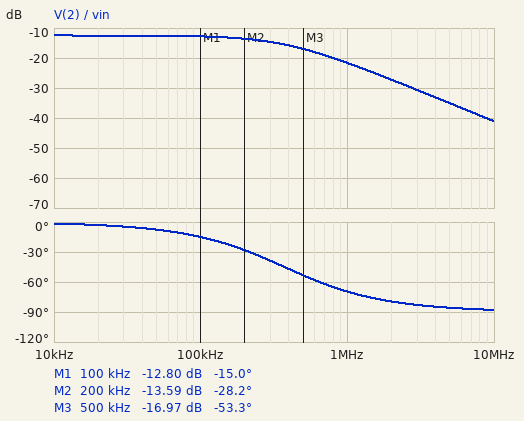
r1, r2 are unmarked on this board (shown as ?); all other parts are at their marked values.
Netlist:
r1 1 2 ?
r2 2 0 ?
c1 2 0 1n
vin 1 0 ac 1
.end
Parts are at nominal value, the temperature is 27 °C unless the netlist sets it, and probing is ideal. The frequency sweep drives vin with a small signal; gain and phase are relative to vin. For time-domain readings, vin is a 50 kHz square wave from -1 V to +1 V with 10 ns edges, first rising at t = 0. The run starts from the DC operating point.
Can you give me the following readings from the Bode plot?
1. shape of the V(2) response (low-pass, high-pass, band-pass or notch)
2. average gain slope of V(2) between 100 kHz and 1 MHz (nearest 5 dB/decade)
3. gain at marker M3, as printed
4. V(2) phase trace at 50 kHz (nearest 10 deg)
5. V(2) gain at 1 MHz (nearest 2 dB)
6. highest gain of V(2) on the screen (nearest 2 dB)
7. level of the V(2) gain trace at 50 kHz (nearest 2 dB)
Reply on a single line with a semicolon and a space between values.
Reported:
low-pass; -10 dB/decade; -16.97 dB; -10 deg; -22 dB; -12 dB; -12 dB
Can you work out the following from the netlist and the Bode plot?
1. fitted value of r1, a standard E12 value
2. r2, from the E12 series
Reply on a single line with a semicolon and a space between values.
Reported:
1.8 kΩ; 560 Ω
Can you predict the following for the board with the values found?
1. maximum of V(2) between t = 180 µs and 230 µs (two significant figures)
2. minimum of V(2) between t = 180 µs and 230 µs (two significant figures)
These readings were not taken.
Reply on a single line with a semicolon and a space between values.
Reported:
240 mV; -240 mV
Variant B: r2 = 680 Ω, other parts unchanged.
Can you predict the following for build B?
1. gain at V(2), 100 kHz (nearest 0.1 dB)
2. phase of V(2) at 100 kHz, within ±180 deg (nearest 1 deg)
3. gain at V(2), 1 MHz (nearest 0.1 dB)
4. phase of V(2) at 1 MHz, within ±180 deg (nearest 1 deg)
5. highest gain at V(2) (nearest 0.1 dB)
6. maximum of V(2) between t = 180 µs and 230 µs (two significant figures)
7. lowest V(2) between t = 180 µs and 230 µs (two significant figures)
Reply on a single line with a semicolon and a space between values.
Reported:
-11.6 dB; -17 deg; -21.5 dB; -72 deg; -11.2 dB; 270 mV; -270 mV
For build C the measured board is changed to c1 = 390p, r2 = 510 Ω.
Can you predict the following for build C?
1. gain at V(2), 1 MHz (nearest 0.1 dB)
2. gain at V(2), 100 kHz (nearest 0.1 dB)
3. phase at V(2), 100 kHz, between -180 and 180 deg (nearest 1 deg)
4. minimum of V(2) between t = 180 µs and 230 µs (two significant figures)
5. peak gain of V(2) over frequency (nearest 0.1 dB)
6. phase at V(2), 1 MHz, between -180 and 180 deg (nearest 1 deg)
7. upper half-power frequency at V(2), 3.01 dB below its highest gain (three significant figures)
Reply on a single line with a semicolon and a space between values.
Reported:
-16.0 dB; -13.2 dB; -6 deg; -220 mV; -13.1 dB; -44 deg; 1.03 MHz
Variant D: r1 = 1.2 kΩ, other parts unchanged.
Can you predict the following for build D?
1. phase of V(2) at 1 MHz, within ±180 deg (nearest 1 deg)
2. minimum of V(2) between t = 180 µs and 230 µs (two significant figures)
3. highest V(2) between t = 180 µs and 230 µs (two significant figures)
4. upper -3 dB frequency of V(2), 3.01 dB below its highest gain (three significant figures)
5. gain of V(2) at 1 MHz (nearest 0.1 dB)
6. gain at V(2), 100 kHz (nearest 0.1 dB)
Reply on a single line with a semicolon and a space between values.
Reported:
-67 deg; -320 mV; 320 mV; 417 kHz; -18.2 dB; -10.2 dB
